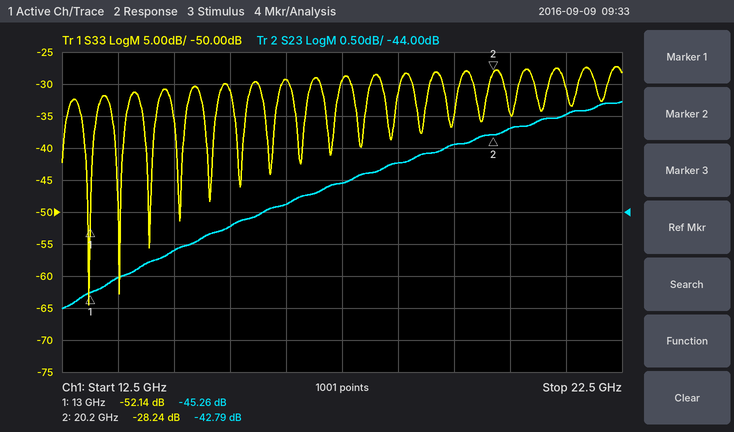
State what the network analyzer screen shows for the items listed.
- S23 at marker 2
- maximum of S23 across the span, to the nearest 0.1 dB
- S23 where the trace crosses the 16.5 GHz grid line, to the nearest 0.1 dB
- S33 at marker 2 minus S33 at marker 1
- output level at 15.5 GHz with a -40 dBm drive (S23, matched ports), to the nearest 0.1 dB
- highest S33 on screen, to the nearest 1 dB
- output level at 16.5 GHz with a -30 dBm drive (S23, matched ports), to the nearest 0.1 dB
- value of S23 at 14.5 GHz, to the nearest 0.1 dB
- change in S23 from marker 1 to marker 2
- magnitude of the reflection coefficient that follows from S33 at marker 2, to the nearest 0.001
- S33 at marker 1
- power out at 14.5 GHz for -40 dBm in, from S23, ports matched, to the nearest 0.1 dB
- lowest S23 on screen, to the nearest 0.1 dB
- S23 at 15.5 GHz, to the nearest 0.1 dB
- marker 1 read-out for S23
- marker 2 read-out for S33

-42.79 dB
-42.3 dB
-43.9 dB
23.90 dB
-84.2 dBm
-27 dB
-73.9 dBm
-44.6 dB
2.47 dB
0.039
-52.14 dB
-84.6 dBm
-45.5 dB
-44.2 dB
-45.26 dB
-28.24 dB
